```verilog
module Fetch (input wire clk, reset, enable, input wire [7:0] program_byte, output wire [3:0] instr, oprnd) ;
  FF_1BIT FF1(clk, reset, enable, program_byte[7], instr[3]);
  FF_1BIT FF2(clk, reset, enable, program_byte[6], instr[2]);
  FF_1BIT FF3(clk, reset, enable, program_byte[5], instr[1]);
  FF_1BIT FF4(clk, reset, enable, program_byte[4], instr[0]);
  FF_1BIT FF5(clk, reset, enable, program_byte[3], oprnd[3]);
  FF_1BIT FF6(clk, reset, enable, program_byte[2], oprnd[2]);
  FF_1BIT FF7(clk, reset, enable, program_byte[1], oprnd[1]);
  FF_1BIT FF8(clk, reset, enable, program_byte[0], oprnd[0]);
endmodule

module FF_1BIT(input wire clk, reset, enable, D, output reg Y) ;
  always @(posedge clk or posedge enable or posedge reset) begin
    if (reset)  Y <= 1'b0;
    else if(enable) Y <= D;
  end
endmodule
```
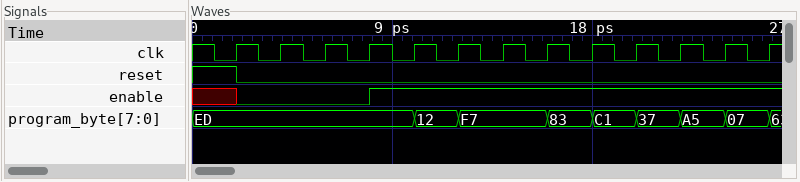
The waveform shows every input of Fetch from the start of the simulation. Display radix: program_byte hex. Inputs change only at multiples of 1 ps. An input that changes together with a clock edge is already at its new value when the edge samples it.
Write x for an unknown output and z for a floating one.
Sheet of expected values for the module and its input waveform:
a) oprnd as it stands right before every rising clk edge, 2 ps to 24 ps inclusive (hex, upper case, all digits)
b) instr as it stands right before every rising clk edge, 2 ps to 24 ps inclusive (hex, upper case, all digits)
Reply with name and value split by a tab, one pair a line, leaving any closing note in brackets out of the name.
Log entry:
oprnd as it stands right before every rising clk edge, 2 ps to 24 ps inclusive	0, 0, 0, 0, D, 2, 7, 7, 3, 1, 7, 5
instr as it stands right before every rising clk edge, 2 ps to 24 ps inclusive	0, 0, 0, 0, E, 1, F, F, 8, C, 3, A
